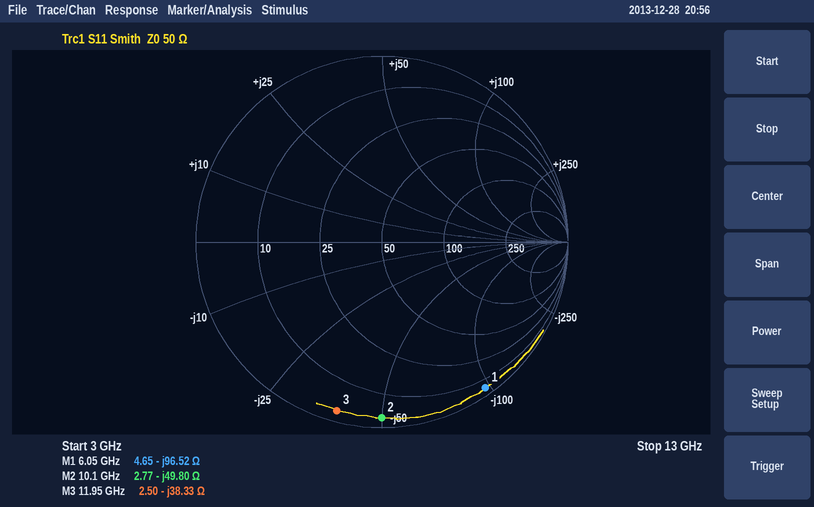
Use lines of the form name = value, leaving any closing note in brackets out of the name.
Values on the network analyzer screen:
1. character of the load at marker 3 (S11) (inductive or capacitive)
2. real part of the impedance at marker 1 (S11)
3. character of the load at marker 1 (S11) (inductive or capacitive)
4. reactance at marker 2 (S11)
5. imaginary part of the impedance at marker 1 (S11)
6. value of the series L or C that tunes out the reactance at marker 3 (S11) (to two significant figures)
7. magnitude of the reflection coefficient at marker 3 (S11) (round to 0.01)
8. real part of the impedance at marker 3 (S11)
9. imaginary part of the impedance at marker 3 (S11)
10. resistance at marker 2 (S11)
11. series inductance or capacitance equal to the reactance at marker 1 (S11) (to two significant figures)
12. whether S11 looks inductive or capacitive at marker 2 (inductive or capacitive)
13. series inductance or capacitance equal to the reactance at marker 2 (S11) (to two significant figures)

character of the load at marker 3 (S11) = capacitive
real part of the impedance at marker 1 = 4.65 Ω
character of the load at marker 1 (S11) = capacitive
reactance at marker 2 = -49.80 Ω
imaginary part of the impedance at marker 1 = -96.52 Ω
value of the series L or C that tunes out the reactance at marker 3 (S11) = 510 pH
magnitude of the reflection coefficient at marker 3 (S11) = 0.94
real part of the impedance at marker 3 = 2.50 Ω
imaginary part of the impedance at marker 3 = -38.33 Ω
resistance at marker 2 = 2.77 Ω
series inductance or capacitance equal to the reactance at marker 1 (S11) = 270 fF
whether S11 looks inductive or capacitive at marker 2 = capacitive
series inductance or capacitance equal to the reactance at marker 2 (S11) = 320 fF
